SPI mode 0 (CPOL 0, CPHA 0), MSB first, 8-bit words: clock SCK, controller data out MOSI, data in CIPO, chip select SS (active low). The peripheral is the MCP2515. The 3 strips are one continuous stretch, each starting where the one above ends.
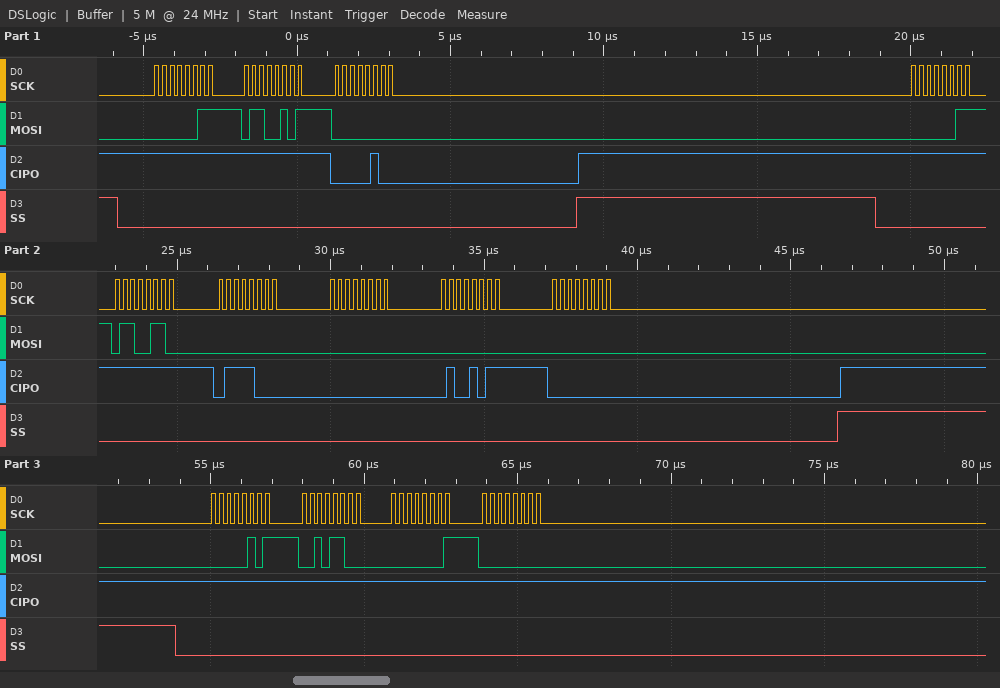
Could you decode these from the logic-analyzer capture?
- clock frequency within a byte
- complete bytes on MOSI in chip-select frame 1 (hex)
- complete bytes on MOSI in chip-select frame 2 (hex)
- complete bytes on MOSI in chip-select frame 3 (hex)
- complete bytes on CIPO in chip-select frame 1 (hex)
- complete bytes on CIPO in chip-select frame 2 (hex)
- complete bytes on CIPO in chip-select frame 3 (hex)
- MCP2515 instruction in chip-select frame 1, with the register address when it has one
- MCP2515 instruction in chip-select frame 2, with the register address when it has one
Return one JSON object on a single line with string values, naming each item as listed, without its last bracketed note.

{"clock frequency within a byte": "4 MHz", "complete bytes on MOSI in chip-select frame 1": "03 65 00", "complete bytes on MOSI in chip-select frame 2": "03 66 00 00 00 00", "complete bytes on MOSI in chip-select frame 3": "05 2C 01 00", "complete bytes on CIPO in chip-select frame 1": "FF FF 04", "complete bytes on CIPO in chip-select frame 2": "FF FF 78 00 4B 00", "complete bytes on CIPO in chip-select frame 3": "FF FF FF FF", "MCP2515 instruction in chip-select frame 1, with the register address when it has one": "READ 0x65", "MCP2515 instruction in chip-select frame 2, with the register address when it has one": "READ 0x66"}
